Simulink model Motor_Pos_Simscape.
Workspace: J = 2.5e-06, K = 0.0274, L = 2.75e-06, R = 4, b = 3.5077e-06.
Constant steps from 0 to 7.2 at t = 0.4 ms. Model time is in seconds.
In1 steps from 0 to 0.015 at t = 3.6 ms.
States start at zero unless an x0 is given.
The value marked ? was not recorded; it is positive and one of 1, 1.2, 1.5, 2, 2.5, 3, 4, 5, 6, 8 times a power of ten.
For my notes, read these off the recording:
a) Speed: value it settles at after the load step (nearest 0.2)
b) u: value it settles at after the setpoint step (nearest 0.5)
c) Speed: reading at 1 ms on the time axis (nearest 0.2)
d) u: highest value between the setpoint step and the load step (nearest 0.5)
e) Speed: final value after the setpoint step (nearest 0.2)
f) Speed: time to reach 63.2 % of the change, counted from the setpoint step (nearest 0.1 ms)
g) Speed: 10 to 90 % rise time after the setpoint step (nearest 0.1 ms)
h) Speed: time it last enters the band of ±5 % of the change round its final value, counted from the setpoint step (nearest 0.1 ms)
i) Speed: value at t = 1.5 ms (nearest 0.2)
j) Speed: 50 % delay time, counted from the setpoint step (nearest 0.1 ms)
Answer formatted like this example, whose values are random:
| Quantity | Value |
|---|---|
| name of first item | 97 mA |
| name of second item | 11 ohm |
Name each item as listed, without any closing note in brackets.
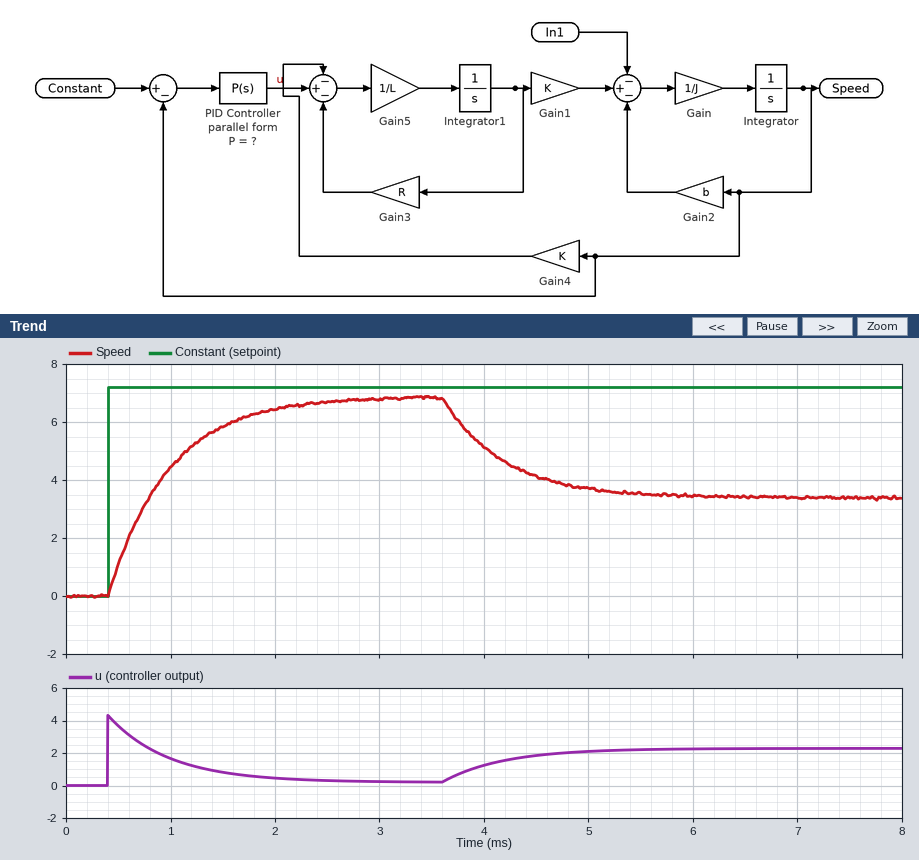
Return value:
| Quantity | Value |
|---|---|
| Speed: value it settles at after the load step | 3.4 |
| u: value it settles at after the setpoint step | 0.0 |
| Speed: reading at 1 ms on the time axis | 4.4 |
| u: highest value between the setpoint step and the load step | 4.5 |
| Speed: final value after the setpoint step | 6.8 |
| Speed: time to reach 63.2 % of the change, counted from the setpoint step | 0.6 ms |
| Speed: 10 to 90 % rise time after the setpoint step | 1.3 ms |
| Speed: time it last enters the band of ±5 % of the change round its final value, counted from the setpoint step | 1.7 ms |
| Speed: value at t = 1.5 ms | 5.8 |
| Speed: 50 % delay time, counted from the setpoint step | 0.4 ms |
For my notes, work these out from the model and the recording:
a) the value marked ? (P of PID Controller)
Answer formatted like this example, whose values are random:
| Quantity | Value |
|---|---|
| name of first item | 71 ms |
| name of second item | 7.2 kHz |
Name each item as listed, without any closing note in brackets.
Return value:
| Quantity | Value |
|---|---|
| the value marked ? | 0.6 |
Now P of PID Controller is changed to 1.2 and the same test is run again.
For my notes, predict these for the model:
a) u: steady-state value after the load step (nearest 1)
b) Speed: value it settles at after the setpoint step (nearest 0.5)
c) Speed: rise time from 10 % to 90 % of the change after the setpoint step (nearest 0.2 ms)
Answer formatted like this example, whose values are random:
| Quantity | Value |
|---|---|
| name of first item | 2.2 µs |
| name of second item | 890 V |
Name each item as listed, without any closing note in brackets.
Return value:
| Quantity | Value |
|---|---|
| u: steady-state value after the load step | 2 |
| Speed: value it settles at after the setpoint step | 7.0 |
| Speed: rise time from 10 % to 90 % of the change after the setpoint step | 0.6 ms |
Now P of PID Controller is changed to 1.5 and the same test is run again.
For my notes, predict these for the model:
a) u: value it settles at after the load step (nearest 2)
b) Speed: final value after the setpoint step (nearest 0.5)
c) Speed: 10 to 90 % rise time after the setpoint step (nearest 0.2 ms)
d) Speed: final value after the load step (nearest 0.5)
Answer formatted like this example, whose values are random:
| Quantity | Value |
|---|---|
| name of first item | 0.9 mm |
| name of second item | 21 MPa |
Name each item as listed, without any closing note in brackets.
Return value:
| Quantity | Value |
|---|---|
| u: value it settles at after the load step | 2 |
| Speed: final value after the setpoint step | 7.0 |
| Speed: 10 to 90 % rise time after the setpoint step | 0.6 ms |
| Speed: final value after the load step | 5.5 |
